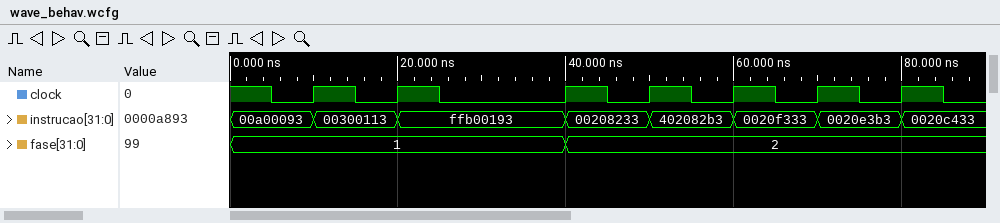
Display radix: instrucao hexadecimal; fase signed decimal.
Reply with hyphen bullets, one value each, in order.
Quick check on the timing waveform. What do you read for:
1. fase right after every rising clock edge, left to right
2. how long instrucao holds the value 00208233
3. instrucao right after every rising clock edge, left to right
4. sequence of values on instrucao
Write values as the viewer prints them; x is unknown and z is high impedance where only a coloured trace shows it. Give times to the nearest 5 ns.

- 1, 1, 2, 2, 2, 2, 2
- 10 ns
- 00300113, ffb00193, 00208233, 402082b3, 0020f333, 0020e3b3, 0020c433
- 00a00093, 00300113, ffb00193, 00208233, 402082b3, 0020f333, 0020e3b3, 0020c433
